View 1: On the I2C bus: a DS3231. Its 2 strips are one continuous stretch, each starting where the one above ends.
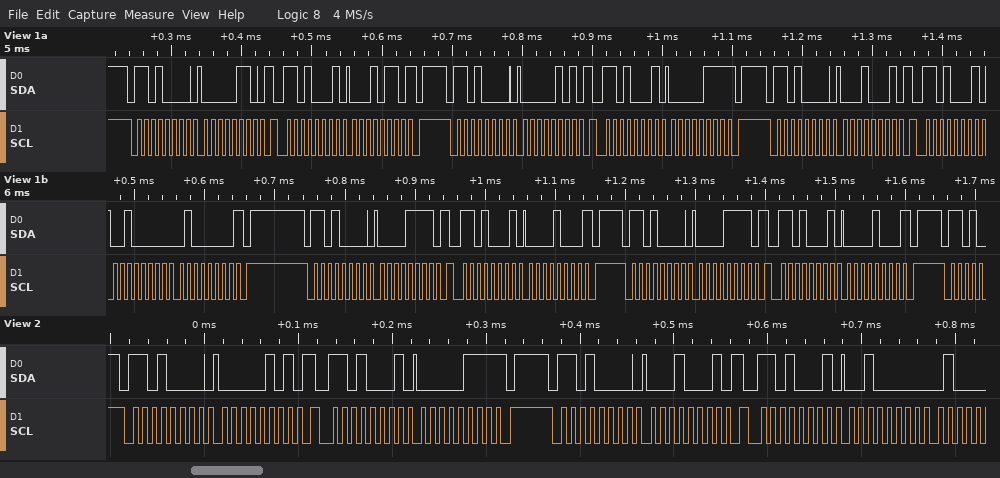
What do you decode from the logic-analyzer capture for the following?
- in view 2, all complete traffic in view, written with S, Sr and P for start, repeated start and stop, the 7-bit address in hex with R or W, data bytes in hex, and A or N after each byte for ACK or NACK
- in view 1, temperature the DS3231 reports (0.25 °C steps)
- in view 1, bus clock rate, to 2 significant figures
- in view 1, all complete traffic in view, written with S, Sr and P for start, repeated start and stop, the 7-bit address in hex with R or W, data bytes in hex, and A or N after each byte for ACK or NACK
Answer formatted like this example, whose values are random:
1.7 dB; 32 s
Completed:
S 68W A 05 A Sr 68R A 07 N P S 68W A 11 A Sr 68R A 20 A; 32.25 °C; 100 kHz; S 68W A 06 A Sr 68R A 16 N P S 68W A 05 A Sr 68R A 07 N P S 68W A 11 A Sr 68R A 20 A 40 N P S 68W A 0F A Sr 68R A 08 N P S 68W A 0F A Sr 68R A 08 N P
